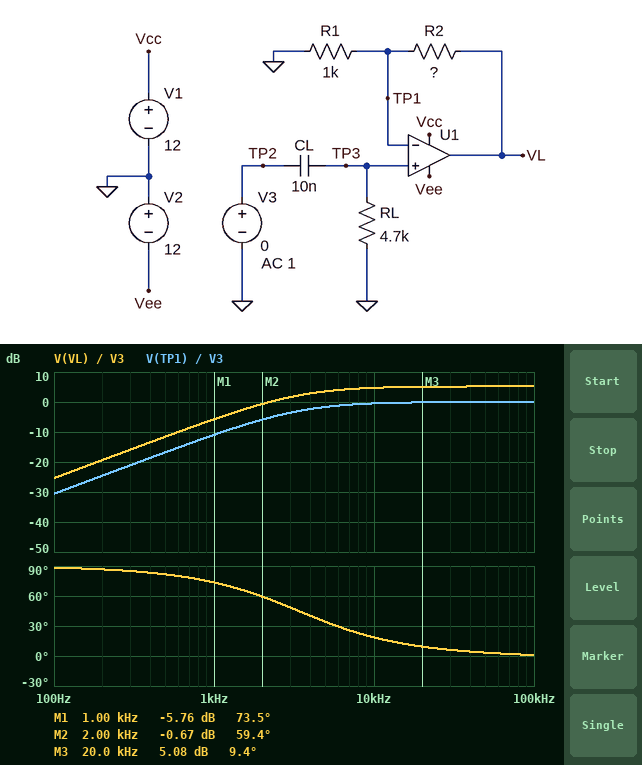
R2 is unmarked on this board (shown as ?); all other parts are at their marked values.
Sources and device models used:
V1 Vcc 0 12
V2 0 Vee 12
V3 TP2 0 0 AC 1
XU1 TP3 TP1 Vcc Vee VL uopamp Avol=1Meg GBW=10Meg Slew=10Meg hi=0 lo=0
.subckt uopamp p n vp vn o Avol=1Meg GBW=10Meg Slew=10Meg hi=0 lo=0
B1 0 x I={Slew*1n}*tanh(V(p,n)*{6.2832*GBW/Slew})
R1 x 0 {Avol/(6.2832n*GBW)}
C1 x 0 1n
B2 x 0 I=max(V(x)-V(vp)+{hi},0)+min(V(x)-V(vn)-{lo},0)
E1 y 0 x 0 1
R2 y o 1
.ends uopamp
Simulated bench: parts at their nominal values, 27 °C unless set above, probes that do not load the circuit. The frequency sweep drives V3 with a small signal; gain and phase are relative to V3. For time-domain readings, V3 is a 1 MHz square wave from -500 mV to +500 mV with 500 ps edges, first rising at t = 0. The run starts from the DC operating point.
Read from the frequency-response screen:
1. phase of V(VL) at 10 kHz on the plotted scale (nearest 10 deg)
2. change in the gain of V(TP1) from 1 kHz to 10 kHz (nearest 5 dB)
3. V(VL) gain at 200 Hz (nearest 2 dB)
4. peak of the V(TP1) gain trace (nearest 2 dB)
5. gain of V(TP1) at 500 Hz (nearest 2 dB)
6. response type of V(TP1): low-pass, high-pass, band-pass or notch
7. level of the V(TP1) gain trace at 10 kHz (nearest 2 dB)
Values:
20 deg
10 dB
-20 dB
0 dB
-16 dB
high-pass
0 dB
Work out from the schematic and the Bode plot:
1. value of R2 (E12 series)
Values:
820 Ω
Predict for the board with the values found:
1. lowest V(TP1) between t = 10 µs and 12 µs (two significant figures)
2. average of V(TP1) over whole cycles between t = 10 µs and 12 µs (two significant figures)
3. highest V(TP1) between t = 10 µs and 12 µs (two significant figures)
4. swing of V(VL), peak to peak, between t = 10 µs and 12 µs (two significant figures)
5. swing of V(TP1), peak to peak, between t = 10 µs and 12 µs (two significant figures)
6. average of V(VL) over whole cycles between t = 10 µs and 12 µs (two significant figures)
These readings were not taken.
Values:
-110 mV
400 mV
900 mV
1.8 V
1.0 V
720 mV
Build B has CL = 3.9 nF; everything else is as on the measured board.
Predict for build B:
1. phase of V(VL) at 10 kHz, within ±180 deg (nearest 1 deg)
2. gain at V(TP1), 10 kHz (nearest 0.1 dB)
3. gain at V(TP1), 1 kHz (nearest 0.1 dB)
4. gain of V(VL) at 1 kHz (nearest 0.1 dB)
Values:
41 deg
-2.4 dB
-18.8 dB
-13.6 dB
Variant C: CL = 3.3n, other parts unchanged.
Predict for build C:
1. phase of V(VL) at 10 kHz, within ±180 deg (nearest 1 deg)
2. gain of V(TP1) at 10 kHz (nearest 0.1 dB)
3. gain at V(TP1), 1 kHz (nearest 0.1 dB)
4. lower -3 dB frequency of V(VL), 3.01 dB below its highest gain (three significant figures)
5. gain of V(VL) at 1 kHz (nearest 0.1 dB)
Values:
46 deg
-3.1 dB
-20.3 dB
10.2 kHz
-15.1 dB
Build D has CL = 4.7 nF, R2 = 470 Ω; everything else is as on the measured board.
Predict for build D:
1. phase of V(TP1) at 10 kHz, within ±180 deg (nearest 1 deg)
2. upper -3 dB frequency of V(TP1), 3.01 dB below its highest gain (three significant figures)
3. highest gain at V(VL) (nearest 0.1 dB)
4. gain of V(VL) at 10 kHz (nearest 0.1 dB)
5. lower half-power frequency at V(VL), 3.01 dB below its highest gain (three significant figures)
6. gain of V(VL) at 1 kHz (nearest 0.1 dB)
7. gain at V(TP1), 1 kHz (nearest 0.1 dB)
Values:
36 deg
6.81 MHz
3.3 dB
1.5 dB
7.19 kHz
-13.9 dB
-17.2 dB
